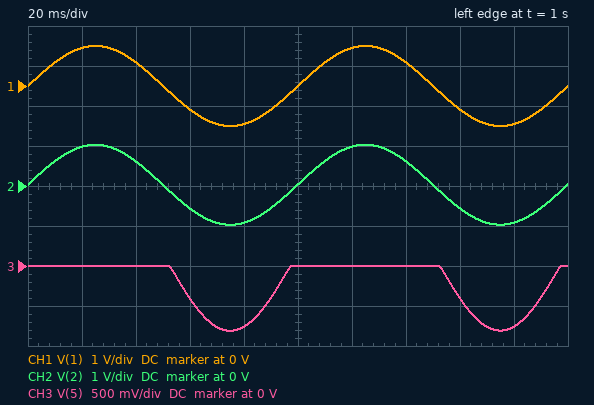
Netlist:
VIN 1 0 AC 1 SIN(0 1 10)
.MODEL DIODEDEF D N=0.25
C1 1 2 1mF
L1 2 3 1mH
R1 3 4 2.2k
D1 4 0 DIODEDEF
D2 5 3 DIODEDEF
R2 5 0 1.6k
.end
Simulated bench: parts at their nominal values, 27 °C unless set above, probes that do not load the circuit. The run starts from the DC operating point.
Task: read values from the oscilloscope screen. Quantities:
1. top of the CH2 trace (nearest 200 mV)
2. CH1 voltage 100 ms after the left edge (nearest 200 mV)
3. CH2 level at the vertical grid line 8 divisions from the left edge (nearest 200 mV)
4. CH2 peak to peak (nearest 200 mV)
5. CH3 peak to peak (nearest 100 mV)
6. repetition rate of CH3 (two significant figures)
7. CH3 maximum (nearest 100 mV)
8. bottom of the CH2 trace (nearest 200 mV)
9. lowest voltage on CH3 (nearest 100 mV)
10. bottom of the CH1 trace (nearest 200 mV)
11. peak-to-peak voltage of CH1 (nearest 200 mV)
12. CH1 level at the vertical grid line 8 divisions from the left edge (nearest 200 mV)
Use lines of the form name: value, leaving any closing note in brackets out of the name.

top of the CH2 trace: 1.0 V
CH1 voltage 100 ms after the left edge: 0 V
CH2 level at the vertical grid line 8 divisions from the left edge: -600 mV
CH2 peak to peak: 2.0 V
CH3 peak to peak: 800 mV
repetition rate of CH3: 10 Hz
CH3 maximum: 0 V
bottom of the CH2 trace: -1.0 V
lowest voltage on CH3: -800 mV
bottom of the CH1 trace: -1.0 V
peak-to-peak voltage of CH1: 2.0 V
CH1 level at the vertical grid line 8 divisions from the left edge: -600 mV
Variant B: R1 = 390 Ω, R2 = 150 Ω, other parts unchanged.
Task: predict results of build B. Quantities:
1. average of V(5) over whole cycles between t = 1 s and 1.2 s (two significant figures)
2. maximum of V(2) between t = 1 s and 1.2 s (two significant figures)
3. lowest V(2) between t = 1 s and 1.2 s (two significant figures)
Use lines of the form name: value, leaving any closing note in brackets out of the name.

average of V(5) over whole cycles between t = 1 s and 1.2 s: -140 mV
maximum of V(2) between t = 1 s and 1.2 s: 1.2 V
lowest V(2) between t = 1 s and 1.2 s: -760 mV
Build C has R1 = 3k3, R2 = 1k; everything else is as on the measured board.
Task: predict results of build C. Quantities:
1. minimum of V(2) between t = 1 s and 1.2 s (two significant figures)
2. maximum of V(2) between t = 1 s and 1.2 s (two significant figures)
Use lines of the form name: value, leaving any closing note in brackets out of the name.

minimum of V(2) between t = 1 s and 1.2 s: -870 mV
maximum of V(2) between t = 1 s and 1.2 s: 1.1 V
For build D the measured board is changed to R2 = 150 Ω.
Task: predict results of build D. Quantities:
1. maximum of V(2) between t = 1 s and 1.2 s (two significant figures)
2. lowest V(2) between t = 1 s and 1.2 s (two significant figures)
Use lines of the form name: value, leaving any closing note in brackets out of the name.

maximum of V(2) between t = 1 s and 1.2 s: 1.5 V
lowest V(2) between t = 1 s and 1.2 s: -480 mV
